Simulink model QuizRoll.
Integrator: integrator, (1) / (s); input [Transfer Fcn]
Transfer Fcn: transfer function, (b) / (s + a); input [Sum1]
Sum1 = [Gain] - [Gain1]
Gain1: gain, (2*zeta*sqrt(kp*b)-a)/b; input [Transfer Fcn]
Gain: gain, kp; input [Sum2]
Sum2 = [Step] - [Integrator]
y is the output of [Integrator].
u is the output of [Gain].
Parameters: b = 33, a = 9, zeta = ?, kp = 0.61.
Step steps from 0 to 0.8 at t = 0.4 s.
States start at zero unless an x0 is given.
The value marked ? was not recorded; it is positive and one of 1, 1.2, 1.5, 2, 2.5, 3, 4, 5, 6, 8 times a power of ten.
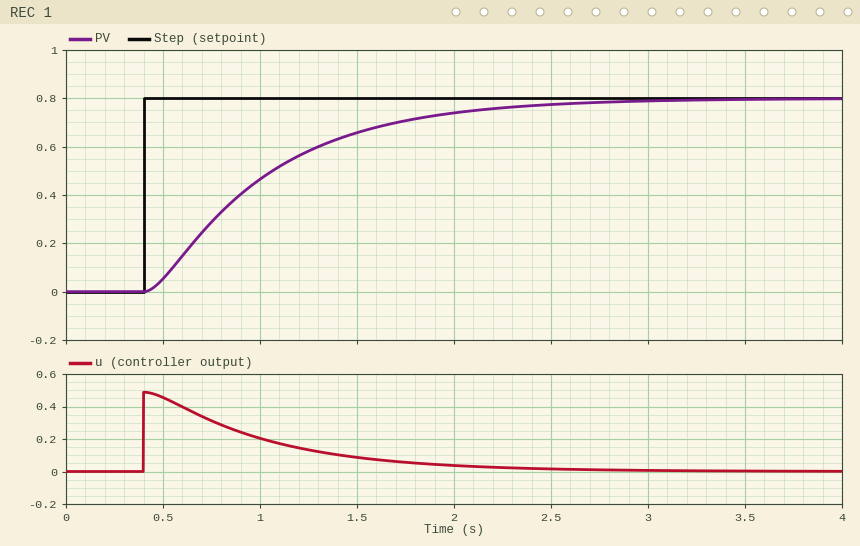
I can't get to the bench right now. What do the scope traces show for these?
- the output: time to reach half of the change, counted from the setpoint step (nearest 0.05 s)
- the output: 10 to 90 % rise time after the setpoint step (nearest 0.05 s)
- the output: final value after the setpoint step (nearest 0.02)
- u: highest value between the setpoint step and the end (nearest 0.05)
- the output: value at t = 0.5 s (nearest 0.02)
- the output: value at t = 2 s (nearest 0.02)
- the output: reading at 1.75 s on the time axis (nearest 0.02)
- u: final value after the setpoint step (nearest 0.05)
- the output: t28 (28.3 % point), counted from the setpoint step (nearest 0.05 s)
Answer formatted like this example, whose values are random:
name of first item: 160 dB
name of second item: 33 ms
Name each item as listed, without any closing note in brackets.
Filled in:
the output: time to reach half of the change, counted from the setpoint step: 0.50 s
the output: 10 to 90 % rise time after the setpoint step: 1.30 s
the output: final value after the setpoint step: 0.80
u: highest value between the setpoint step and the end: 0.50
the output: value at t = 0.5 s: 0.06
the output: value at t = 2 s: 0.74
the output: reading at 1.75 s on the time axis: 0.70
u: final value after the setpoint step: 0.00
the output: t28 (28.3 % point), counted from the setpoint step: 0.30 s
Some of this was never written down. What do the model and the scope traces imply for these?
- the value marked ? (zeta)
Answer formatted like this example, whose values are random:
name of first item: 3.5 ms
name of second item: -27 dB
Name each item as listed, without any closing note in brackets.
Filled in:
the value marked ?: 1.5
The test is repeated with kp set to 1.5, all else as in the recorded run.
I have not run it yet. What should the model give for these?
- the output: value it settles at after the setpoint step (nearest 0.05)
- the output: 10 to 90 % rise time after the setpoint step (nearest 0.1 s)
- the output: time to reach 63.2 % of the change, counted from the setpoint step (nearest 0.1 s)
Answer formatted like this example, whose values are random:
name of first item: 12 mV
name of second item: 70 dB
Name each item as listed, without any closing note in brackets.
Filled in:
the output: value it settles at after the setpoint step: 0.80
the output: 10 to 90 % rise time after the setpoint step: 0.8 s
the output: time to reach 63.2 % of the change, counted from the setpoint step: 0.4 s
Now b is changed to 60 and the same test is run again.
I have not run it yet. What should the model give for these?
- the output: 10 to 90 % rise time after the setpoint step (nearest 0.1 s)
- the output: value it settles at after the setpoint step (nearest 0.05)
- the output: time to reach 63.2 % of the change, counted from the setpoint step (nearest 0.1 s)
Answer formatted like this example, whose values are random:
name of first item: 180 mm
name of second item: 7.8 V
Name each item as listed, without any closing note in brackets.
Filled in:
the output: 10 to 90 % rise time after the setpoint step: 1.0 s
the output: value it settles at after the setpoint step: 0.80
the output: time to reach 63.2 % of the change, counted from the setpoint step: 0.5 s
